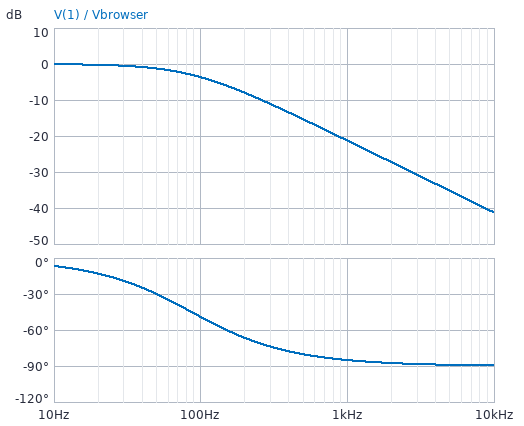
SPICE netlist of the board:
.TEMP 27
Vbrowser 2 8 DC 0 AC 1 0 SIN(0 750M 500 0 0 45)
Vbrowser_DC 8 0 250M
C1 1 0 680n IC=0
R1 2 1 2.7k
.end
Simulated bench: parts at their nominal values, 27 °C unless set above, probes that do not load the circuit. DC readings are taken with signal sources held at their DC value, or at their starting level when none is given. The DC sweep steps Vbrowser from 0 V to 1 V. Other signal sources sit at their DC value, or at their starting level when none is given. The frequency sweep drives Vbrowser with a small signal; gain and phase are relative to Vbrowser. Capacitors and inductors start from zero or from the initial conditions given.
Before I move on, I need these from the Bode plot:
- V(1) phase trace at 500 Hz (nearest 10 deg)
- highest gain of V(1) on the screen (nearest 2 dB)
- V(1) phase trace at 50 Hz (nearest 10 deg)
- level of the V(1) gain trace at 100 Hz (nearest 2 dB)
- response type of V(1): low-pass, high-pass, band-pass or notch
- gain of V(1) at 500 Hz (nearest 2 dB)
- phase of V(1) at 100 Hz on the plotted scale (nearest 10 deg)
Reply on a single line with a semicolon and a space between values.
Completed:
-80 deg; 0 dB; -30 deg; -4 dB; low-pass; -16 dB; -50 deg
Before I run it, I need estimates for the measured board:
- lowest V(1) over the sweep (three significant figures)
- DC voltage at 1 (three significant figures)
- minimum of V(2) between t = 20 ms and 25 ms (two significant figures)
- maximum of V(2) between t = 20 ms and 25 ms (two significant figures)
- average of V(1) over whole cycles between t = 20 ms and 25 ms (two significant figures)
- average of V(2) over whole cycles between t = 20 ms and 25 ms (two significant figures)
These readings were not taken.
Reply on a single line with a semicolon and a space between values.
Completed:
250 mV; 250 mV; -500 mV; 1.0 V; 250 mV; 250 mV
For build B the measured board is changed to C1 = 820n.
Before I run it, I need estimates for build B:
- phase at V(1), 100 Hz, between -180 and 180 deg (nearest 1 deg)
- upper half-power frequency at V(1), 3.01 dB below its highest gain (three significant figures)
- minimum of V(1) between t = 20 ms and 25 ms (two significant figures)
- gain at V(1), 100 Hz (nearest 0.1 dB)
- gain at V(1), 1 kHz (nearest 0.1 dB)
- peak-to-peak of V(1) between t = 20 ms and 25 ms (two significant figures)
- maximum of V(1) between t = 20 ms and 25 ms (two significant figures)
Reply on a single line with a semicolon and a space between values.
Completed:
-54 deg; 71.9 Hz; 140 mV; -4.7 dB; -22.9 dB; 210 mV; 360 mV
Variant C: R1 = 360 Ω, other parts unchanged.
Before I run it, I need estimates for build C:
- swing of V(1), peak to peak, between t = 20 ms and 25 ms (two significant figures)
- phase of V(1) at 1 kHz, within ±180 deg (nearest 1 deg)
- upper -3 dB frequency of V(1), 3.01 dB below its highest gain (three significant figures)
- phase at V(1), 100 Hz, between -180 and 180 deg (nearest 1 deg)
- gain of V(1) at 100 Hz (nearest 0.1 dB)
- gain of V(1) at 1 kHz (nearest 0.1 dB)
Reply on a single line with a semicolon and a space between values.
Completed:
1.2 V; -57 deg; 650 Hz; -9 deg; -0.1 dB; -5.3 dB
